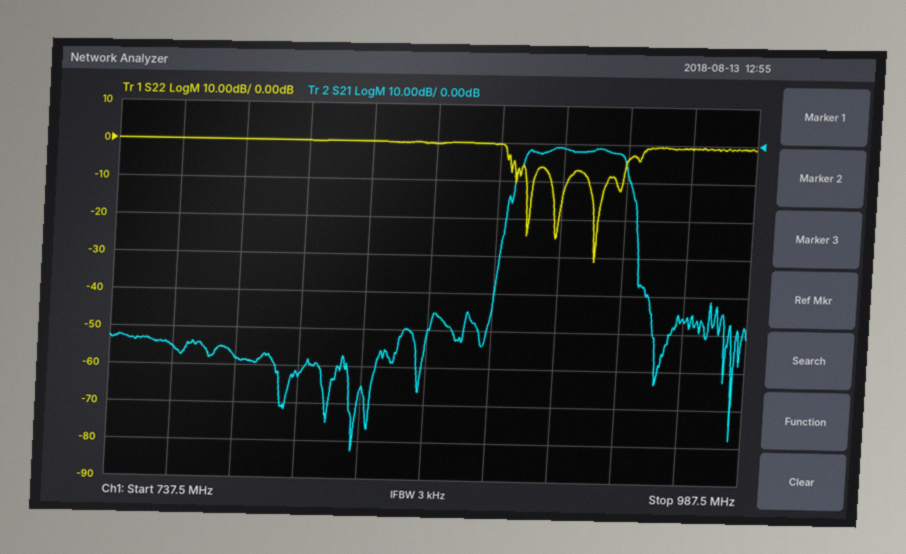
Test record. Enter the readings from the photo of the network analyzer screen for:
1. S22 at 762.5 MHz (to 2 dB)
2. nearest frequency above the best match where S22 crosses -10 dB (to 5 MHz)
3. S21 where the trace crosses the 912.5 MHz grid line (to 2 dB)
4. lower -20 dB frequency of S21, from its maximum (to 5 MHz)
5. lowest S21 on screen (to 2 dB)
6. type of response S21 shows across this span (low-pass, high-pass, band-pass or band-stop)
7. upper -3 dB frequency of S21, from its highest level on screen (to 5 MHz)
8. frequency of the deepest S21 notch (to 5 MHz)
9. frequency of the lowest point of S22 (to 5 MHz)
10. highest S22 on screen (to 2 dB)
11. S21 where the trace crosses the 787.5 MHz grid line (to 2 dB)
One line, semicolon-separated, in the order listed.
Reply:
0 dB; 930 MHz; -2 dB; 890 MHz; -82 dB; band-pass; 935 MHz; 835 MHz; 925 MHz; 0 dB; -58 dB
